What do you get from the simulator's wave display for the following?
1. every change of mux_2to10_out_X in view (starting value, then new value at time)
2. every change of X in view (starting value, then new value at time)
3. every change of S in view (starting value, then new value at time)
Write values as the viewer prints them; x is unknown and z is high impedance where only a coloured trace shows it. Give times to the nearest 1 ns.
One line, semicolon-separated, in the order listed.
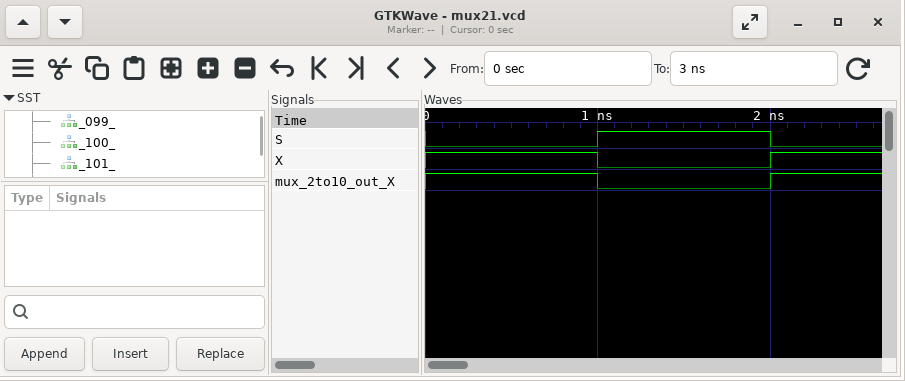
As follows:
1, 0 at 1 ns, 1 at 2 ns; 1, 0 at 1 ns, 1 at 2 ns; 0, 1 at 1 ns, 0 at 2 ns
